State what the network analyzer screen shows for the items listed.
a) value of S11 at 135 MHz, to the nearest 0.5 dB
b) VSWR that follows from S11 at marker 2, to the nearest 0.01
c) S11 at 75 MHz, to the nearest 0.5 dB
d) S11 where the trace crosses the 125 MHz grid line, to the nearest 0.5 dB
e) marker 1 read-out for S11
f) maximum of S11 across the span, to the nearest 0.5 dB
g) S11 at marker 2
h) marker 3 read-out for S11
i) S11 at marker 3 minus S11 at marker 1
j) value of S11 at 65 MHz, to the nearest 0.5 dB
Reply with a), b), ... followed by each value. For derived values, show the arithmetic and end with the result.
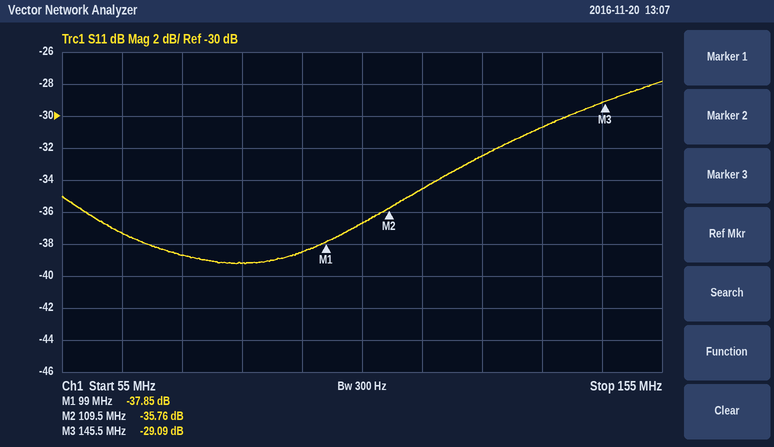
a) -30.5 dB
b) (1 + 0.0163)/(1 − 0.0163) ≈ 1.03
c) -38.5 dB
d) -32.5 dB
e) -37.85 dB
f) -28.0 dB
g) -35.76 dB
h) -29.09 dB
i) -29.09 − (-37.85) = 8.76 dB
j) -37.5 dB
